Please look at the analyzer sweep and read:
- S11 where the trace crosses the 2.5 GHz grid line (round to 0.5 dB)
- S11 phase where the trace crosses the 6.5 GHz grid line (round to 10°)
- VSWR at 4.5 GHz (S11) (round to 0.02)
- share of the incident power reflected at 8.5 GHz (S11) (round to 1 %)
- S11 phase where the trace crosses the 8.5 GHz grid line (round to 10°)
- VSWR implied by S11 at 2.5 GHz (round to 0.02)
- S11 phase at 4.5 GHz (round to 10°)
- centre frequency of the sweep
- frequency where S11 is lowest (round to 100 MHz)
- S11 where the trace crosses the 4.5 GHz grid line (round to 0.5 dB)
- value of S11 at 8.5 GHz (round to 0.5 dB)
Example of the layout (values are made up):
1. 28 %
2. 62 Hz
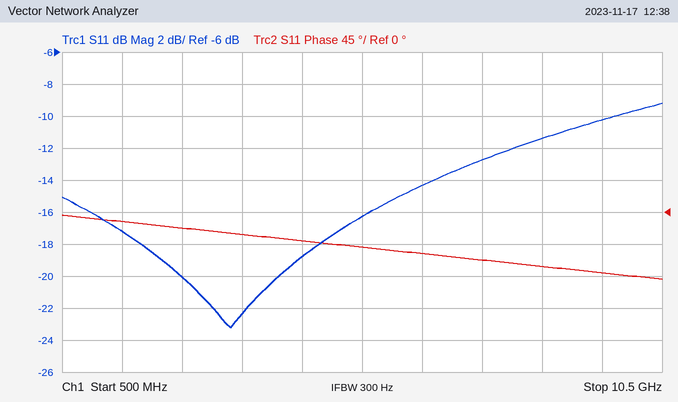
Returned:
1. -20.0 dB
2. -60°
3. 1.26
4. 7 %
5. -80°
6. 1.22
7. -40°
8. 5.5 GHz
9. 3.3 GHz
10. -19.0 dB
11. -11.5 dB
